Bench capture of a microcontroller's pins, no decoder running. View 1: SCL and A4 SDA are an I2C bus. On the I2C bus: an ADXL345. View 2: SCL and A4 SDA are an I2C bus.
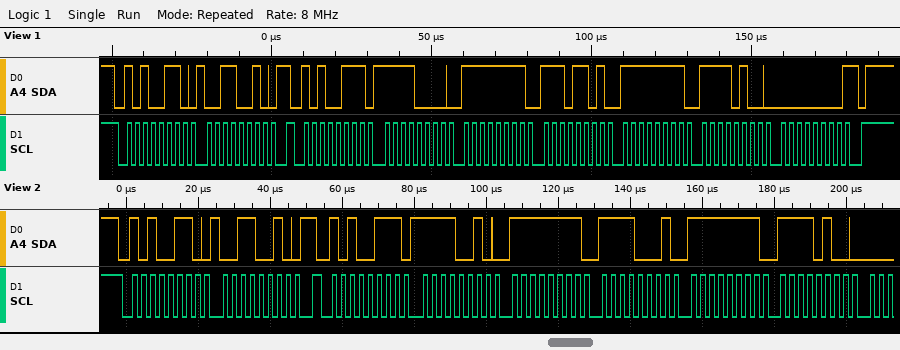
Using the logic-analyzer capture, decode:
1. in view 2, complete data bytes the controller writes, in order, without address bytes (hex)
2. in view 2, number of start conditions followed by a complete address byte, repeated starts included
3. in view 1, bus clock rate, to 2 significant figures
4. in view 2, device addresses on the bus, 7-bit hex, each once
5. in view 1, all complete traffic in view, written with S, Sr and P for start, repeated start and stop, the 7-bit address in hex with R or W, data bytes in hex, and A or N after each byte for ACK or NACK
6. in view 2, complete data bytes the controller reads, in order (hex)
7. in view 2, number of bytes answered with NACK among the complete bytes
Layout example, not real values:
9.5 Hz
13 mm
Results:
32
2
400 kHz
0x53
S 53W A 32 A Sr 53R A F0 A FF A ED A FF A F4 A 00 N P
F2 FF F1 FF F4
0
